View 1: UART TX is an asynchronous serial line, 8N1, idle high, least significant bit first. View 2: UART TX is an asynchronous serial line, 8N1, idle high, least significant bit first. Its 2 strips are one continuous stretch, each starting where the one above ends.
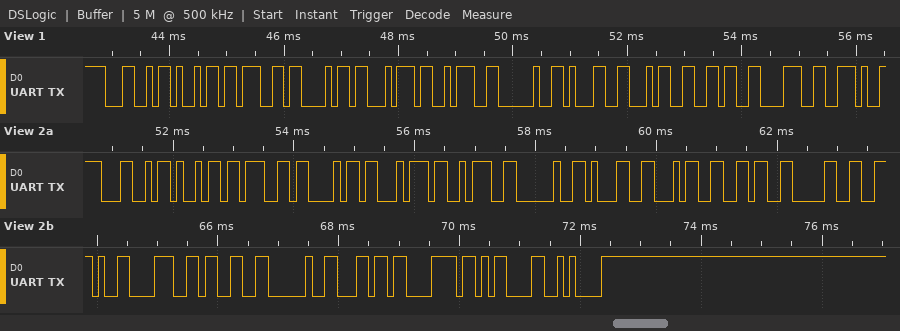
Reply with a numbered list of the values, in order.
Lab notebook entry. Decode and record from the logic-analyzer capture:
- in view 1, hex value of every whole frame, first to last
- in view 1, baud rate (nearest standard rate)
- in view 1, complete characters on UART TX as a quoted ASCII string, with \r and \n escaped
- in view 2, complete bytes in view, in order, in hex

1. 4C 69 67 68 74 3A 20 31 34 36 38 2E
2. 9600 baud
3. "Light: 1468."
4. 4C 69 67 68 74 3A 20 31 34 36 30 2E 38 33 20 6C 78 0D 0A
